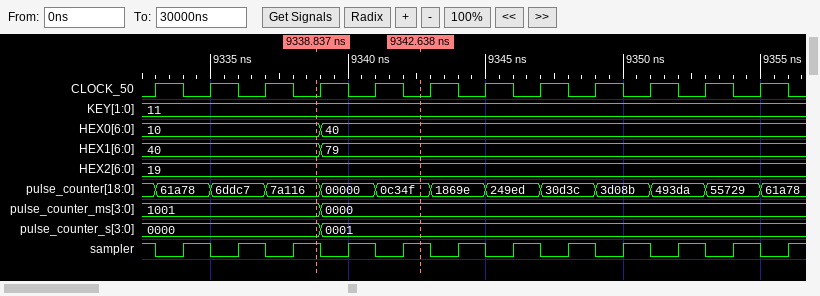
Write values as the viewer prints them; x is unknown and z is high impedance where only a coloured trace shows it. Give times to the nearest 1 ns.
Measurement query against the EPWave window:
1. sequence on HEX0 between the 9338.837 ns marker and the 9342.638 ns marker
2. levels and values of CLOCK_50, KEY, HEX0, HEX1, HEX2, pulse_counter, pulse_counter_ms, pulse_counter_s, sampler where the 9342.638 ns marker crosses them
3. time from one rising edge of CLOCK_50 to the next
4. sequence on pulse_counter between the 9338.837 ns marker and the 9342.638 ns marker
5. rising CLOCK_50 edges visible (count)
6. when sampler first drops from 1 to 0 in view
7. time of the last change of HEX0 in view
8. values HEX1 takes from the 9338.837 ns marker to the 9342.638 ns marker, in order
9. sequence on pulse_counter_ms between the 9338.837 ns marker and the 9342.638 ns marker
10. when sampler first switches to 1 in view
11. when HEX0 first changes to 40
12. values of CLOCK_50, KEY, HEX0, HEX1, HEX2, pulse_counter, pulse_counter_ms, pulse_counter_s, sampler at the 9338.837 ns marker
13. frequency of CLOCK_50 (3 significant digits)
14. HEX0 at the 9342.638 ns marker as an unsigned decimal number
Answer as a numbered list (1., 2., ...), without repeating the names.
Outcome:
1. 10, 40
2. CLOCK_50=0, KEY=11, HEX0=40, HEX1=79, HEX2=19, pulse_counter=0c34f, pulse_counter_ms=0000, pulse_counter_s=0001, sampler=1
3. 2 ns
4. 7a116, 00000, 0c34f
5. 12
6. 9333 ns
7. 9339 ns
8. 40, 79
9. 1001, 0000
10. 9334 ns
11. 9339 ns
12. CLOCK_50=0, KEY=11, HEX0=10, HEX1=40, HEX2=19, pulse_counter=7a116, pulse_counter_ms=1001, pulse_counter_s=0000, sampler=1
13. 500 MHz
14. 64
